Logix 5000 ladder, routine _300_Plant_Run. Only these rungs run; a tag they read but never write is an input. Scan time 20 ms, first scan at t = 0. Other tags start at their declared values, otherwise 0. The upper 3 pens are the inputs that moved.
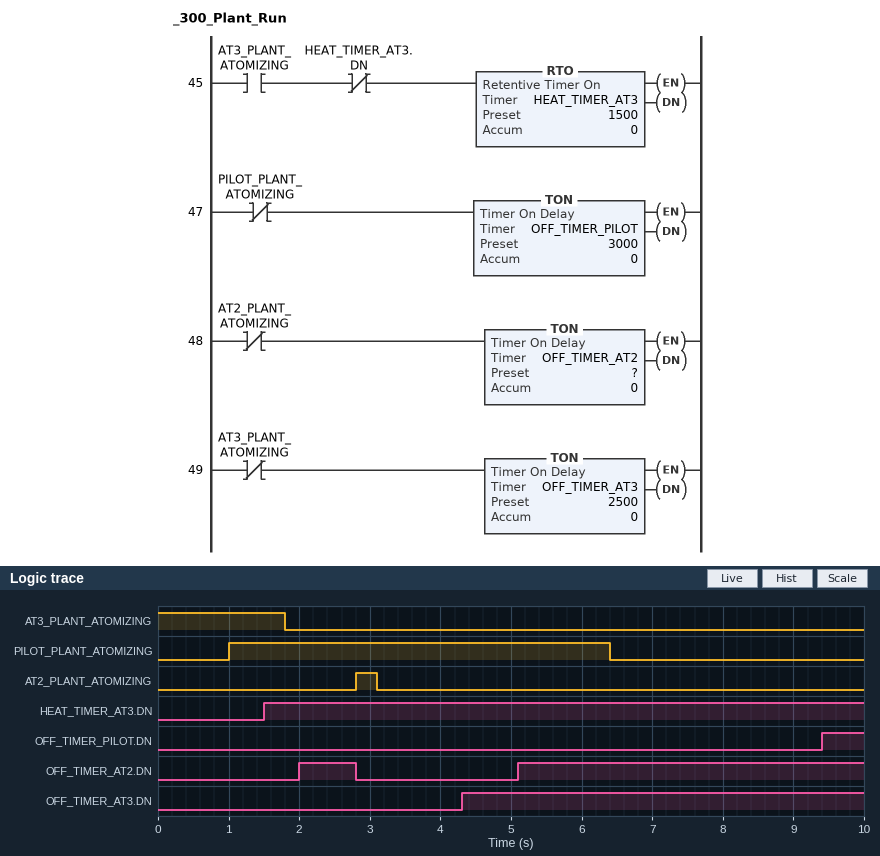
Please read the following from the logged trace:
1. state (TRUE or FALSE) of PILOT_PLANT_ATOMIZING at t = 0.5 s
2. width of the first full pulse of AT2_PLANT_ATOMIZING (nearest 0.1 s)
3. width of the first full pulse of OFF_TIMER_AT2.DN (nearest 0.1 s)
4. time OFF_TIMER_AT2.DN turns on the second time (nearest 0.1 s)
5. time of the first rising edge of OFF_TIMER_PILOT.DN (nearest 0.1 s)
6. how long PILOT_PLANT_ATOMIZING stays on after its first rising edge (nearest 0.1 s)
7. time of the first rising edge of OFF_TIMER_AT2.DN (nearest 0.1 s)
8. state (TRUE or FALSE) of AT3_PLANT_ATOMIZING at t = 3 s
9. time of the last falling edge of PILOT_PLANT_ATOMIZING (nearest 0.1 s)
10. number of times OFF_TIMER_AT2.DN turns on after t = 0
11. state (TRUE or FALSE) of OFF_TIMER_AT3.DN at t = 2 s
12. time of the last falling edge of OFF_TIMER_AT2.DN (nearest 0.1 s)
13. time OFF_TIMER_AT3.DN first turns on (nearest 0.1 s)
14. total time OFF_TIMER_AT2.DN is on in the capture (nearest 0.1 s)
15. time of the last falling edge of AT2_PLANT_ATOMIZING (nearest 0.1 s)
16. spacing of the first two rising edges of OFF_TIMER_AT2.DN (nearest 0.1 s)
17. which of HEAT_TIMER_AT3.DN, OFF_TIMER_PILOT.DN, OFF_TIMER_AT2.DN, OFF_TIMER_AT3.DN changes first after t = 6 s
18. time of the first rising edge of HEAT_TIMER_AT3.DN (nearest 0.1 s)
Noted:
FALSE
0.3 s
0.8 s
5.1 s
9.4 s
5.4 s
2.0 s
FALSE
6.4 s
2
FALSE
2.8 s
4.3 s
5.7 s
3.1 s
3.1 s
OFF_TIMER_PILOT.DN
1.5 s
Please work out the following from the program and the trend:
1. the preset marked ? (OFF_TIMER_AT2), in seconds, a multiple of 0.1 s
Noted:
2.0 s
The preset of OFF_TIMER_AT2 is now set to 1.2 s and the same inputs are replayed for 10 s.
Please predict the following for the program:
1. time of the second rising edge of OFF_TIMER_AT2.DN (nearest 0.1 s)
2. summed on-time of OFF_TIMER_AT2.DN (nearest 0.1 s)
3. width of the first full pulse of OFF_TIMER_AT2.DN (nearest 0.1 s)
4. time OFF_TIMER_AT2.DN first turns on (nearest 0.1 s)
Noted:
4.3 s
7.3 s
1.6 s
1.2 s
